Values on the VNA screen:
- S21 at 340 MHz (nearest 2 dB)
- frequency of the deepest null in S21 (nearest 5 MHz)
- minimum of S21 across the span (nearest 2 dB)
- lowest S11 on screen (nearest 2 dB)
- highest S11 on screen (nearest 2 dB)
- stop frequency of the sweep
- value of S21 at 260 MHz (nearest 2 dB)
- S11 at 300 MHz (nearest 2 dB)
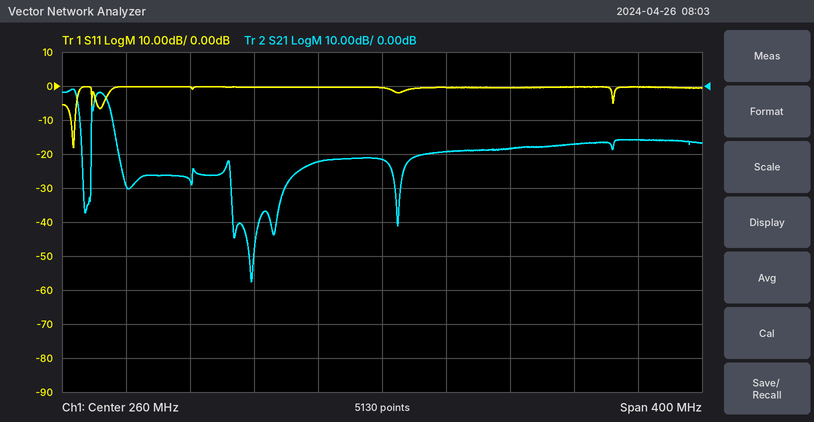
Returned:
-18 dB
180 MHz
-58 dB
-18 dB
0 dB
460 MHz
-22 dB
0 dB
